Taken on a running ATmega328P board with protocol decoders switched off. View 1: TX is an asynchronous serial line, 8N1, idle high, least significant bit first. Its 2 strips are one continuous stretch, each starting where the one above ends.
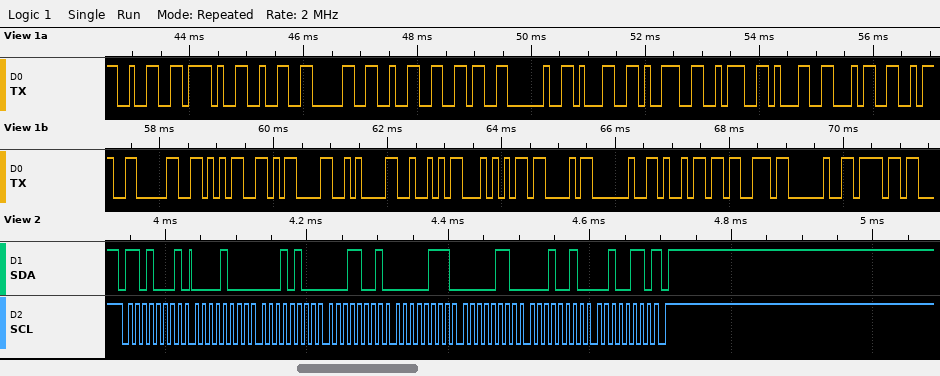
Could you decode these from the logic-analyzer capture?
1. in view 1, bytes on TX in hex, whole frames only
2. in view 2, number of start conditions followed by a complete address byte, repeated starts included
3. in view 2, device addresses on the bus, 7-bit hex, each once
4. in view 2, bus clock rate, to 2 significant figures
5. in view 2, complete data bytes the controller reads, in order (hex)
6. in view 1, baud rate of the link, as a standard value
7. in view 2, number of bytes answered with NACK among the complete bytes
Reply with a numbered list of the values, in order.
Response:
1. 32 2F 32 30 32 36 20 31 39 3A 31 34 3A 30 35 0D 0A 52 54 43 20 69 73 20 6F
2. 1
3. 0x68
4. 100 kHz
5. 08 14 19 07 06 12 26
6. 9600 baud
7. 1
